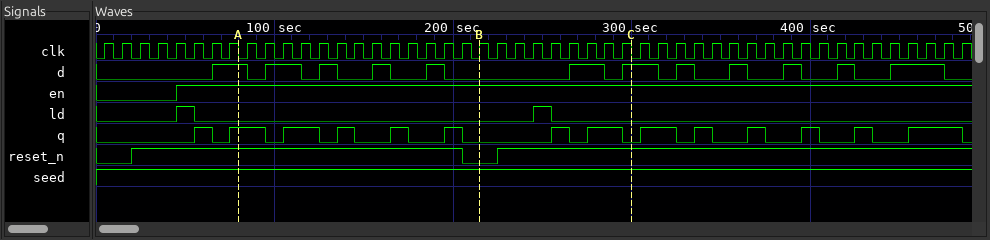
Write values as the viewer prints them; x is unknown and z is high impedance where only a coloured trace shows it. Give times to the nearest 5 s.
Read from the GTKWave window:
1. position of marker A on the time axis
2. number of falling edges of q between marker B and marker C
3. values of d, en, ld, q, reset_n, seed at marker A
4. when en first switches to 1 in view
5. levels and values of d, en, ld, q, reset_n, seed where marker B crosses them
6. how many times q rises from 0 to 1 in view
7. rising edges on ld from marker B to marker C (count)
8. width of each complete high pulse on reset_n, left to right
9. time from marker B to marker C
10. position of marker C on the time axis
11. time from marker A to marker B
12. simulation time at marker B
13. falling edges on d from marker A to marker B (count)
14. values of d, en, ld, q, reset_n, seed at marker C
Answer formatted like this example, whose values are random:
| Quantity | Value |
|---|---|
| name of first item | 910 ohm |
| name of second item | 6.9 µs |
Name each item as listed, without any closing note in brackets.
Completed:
| Quantity | Value |
|---|---|
| position of marker A on the time axis | 80 s |
| number of falling edges of q between marker B and marker C | 2 |
| values of d, en, ld, q, reset_n, seed at marker A | d=1, en=1, ld=0, q=1, reset_n=1, seed=1 |
| when en first switches to 1 in view | 45 s |
| levels and values of d, en, ld, q, reset_n, seed where marker B crosses them | d=0, en=1, ld=0, q=0, reset_n=0, seed=1 |
| how many times q rises from 0 to 1 in view | 14 |
| rising edges on ld from marker B to marker C | 1 |
| width of each complete high pulse on reset_n, left to right | 185 s |
| time from marker B to marker C | 85 s |
| position of marker C on the time axis | 300 s |
| time from marker A to marker B | 135 s |
| simulation time at marker B | 215 s |
| falling edges on d from marker A to marker B | 5 |
| values of d, en, ld, q, reset_n, seed at marker C | d=1, en=1, ld=0, q=0, reset_n=1, seed=1 |
